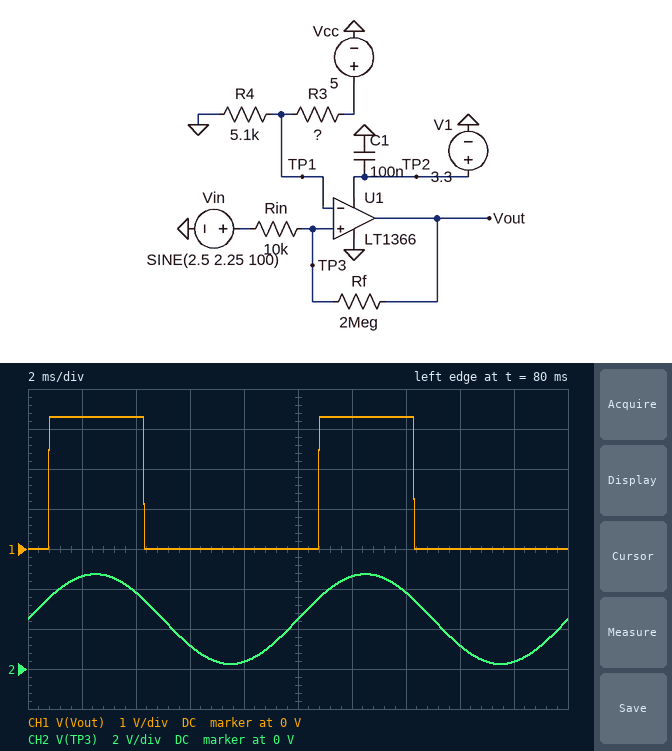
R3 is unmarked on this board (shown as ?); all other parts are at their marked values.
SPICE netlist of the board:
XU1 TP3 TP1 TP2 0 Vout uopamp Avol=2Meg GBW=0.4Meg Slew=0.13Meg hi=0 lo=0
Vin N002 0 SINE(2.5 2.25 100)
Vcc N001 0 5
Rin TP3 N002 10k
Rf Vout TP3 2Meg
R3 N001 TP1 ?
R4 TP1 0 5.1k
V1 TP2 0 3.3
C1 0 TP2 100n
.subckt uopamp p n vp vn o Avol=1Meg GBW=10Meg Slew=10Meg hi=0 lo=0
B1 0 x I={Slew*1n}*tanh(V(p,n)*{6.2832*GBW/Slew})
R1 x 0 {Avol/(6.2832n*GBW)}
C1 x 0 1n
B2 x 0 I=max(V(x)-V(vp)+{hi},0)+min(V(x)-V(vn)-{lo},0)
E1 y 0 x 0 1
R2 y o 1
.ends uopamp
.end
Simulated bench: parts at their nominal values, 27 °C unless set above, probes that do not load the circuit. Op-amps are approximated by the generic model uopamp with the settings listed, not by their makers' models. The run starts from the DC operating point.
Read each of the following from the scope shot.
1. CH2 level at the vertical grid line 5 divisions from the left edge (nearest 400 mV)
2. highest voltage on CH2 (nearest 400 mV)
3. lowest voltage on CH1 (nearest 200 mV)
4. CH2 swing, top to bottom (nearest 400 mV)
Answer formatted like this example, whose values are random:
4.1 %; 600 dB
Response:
2.4 V; 4.8 V; 0 V; 4.4 V
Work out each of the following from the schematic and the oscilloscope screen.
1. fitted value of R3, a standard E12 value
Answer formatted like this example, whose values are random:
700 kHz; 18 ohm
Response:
2.2 kΩ
